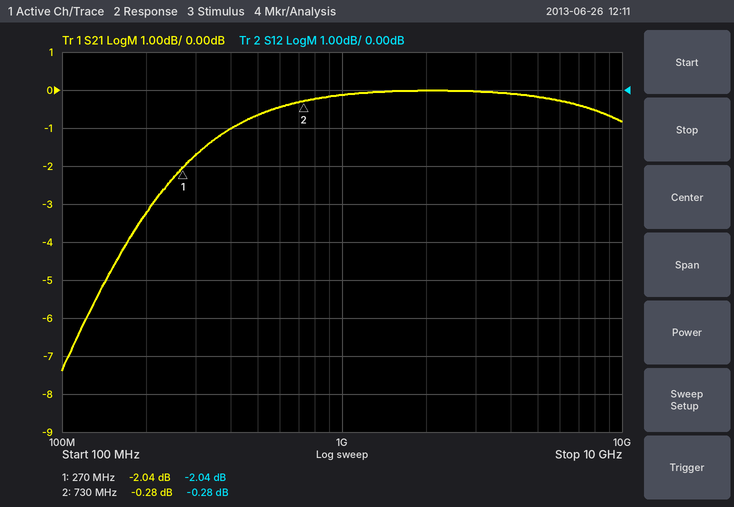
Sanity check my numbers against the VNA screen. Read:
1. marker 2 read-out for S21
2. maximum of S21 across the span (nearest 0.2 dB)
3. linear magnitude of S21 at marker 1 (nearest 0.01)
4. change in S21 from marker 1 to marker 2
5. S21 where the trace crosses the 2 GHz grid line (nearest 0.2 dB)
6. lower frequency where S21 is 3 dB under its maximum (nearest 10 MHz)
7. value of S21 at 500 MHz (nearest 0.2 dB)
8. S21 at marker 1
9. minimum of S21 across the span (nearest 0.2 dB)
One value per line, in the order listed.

-0.28 dB
0.0 dB
0.79
1.76 dB
0.0 dB
210 MHz
-0.6 dB
-2.04 dB
-7.4 dB
